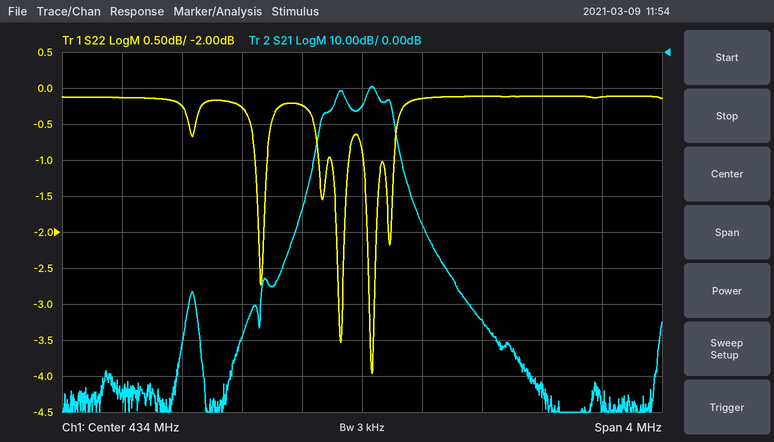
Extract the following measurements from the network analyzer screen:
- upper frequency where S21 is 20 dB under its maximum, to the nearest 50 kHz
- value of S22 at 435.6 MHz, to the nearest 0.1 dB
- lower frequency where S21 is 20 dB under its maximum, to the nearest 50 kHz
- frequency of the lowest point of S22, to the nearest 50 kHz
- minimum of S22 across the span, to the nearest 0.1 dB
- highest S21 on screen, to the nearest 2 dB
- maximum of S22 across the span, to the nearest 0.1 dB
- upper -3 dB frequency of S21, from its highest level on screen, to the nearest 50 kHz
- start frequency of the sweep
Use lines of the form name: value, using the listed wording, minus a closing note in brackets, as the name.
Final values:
upper frequency where S21 is 20 dB under its maximum, to the nearest 50 kHz: 434.25 MHz
value of S22 at 435.6 MHz, to the nearest 0.1 dB: -0.1 dB
lower frequency where S21 is 20 dB under its maximum, to the nearest 50 kHz: 433.70 MHz
frequency of the lowest point of S22, to the nearest 50 kHz: 434.05 MHz
minimum of S22 across the span, to the nearest 0.1 dB: -4.0 dB
highest S21 on screen, to the nearest 2 dB: -10 dB
maximum of S22 across the span, to the nearest 0.1 dB: -0.1 dB
upper -3 dB frequency of S21, from its highest level on screen, to the nearest 50 kHz: 434.10 MHz
start frequency of the sweep: 432 MHz
